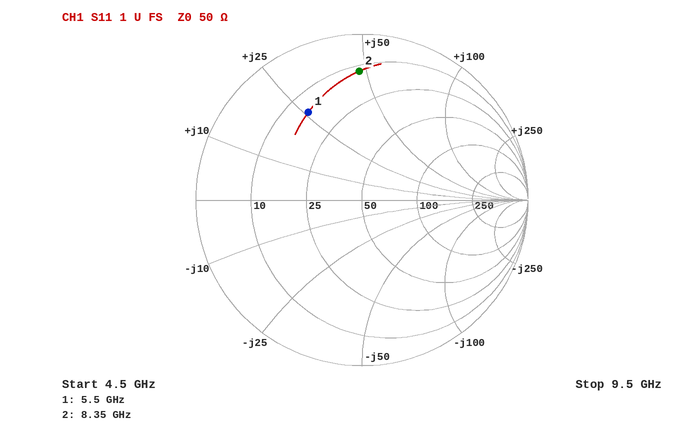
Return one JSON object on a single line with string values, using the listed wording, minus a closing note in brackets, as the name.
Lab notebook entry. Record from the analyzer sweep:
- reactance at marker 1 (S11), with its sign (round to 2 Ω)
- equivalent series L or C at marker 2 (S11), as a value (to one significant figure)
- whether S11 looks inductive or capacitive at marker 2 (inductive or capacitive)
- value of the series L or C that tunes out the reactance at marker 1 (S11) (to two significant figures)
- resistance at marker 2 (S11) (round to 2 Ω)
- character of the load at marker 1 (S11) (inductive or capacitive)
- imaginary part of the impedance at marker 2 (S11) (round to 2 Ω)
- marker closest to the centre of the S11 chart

{"reactance at marker 1 (S11), with its sign": "+26 Ω", "equivalent series L or C at marker 2 (S11), as a value": "900 pH", "whether S11 looks inductive or capacitive at marker 2": "inductive", "value of the series L or C that tunes out the reactance at marker 1 (S11)": "1.1 pF", "resistance at marker 2 (S11)": "12 Ω", "character of the load at marker 1 (S11)": "inductive", "imaginary part of the impedance at marker 2 (S11)": "+48 Ω", "marker closest to the centre of the S11 chart": "marker 1"}
